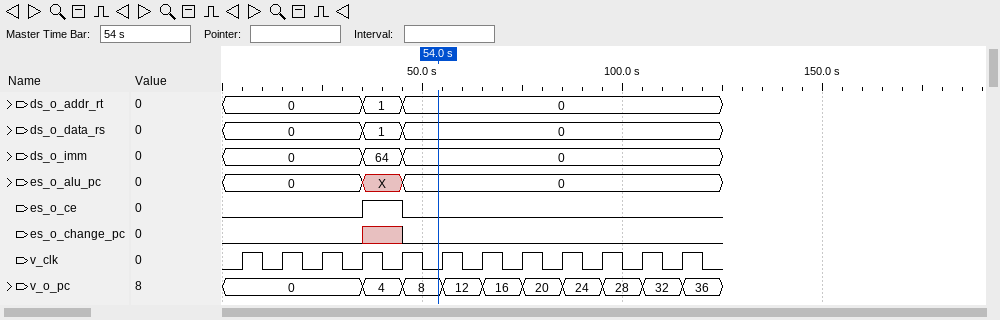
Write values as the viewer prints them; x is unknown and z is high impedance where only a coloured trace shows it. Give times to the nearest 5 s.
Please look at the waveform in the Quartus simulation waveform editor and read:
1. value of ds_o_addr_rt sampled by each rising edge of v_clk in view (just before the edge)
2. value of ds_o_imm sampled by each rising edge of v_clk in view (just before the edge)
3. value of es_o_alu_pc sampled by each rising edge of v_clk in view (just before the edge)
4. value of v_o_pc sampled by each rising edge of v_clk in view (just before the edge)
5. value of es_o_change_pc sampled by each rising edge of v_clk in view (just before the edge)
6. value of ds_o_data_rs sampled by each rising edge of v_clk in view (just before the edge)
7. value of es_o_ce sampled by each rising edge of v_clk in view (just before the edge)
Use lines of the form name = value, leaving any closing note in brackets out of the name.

value of ds_o_addr_rt sampled by each rising edge of v_clk in view = 0, 0, 0, 0, 1, 0, 0, 0, 0, 0, 0, 0
value of ds_o_imm sampled by each rising edge of v_clk in view = 0, 0, 0, 0, 64, 0, 0, 0, 0, 0, 0, 0
value of es_o_alu_pc sampled by each rising edge of v_clk in view = 0, 0, 0, 0, X, 0, 0, 0, 0, 0, 0, 0
value of v_o_pc sampled by each rising edge of v_clk in view = 0, 0, 0, 0, 4, 8, 12, 16, 20, 24, 28, 32
value of es_o_change_pc sampled by each rising edge of v_clk in view = 0 0 0 0 x 0 0 0 0 0 0 0
value of ds_o_data_rs sampled by each rising edge of v_clk in view = 0, 0, 0, 0, 1, 0, 0, 0, 0, 0, 0, 0
value of es_o_ce sampled by each rising edge of v_clk in view = 0 0 0 0 1 0 0 0 0 0 0 0
